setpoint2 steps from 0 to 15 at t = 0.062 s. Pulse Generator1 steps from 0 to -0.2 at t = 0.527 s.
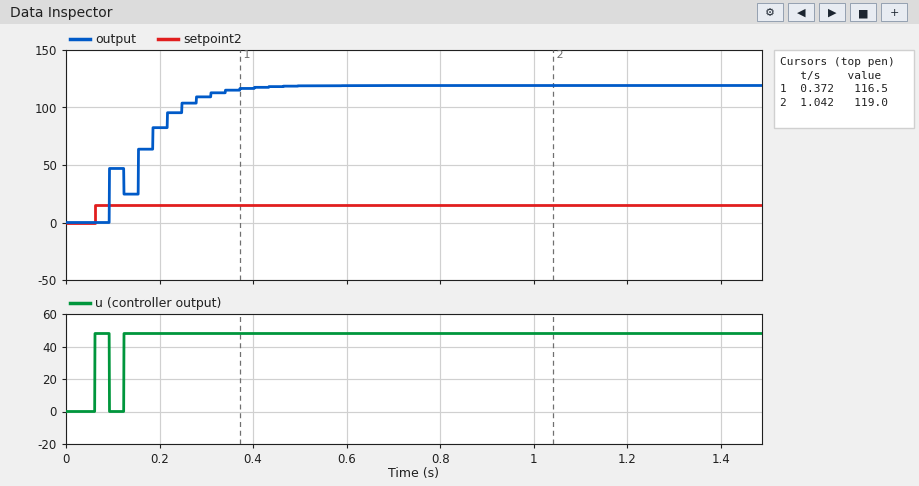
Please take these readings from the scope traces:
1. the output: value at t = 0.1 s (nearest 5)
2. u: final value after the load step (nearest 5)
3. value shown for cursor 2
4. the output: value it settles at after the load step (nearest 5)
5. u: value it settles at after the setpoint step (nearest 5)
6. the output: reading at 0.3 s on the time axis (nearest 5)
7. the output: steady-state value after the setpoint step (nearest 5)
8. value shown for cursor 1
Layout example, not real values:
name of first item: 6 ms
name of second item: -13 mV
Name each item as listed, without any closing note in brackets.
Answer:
the output: value at t = 0.1 s: 45
u: final value after the load step: 50
value shown for cursor 2: 119.0
the output: value it settles at after the load step: 120
u: value it settles at after the setpoint step: 50
the output: reading at 0.3 s on the time axis: 110
the output: steady-state value after the setpoint step: 120
value shown for cursor 1: 116.5
